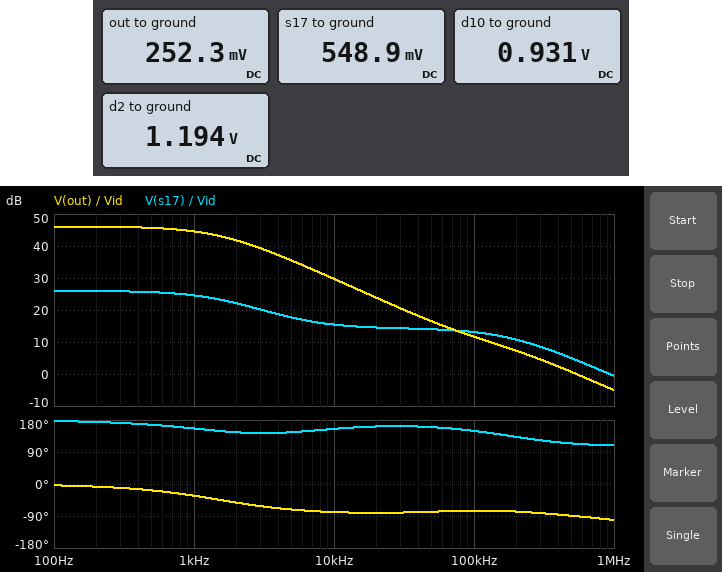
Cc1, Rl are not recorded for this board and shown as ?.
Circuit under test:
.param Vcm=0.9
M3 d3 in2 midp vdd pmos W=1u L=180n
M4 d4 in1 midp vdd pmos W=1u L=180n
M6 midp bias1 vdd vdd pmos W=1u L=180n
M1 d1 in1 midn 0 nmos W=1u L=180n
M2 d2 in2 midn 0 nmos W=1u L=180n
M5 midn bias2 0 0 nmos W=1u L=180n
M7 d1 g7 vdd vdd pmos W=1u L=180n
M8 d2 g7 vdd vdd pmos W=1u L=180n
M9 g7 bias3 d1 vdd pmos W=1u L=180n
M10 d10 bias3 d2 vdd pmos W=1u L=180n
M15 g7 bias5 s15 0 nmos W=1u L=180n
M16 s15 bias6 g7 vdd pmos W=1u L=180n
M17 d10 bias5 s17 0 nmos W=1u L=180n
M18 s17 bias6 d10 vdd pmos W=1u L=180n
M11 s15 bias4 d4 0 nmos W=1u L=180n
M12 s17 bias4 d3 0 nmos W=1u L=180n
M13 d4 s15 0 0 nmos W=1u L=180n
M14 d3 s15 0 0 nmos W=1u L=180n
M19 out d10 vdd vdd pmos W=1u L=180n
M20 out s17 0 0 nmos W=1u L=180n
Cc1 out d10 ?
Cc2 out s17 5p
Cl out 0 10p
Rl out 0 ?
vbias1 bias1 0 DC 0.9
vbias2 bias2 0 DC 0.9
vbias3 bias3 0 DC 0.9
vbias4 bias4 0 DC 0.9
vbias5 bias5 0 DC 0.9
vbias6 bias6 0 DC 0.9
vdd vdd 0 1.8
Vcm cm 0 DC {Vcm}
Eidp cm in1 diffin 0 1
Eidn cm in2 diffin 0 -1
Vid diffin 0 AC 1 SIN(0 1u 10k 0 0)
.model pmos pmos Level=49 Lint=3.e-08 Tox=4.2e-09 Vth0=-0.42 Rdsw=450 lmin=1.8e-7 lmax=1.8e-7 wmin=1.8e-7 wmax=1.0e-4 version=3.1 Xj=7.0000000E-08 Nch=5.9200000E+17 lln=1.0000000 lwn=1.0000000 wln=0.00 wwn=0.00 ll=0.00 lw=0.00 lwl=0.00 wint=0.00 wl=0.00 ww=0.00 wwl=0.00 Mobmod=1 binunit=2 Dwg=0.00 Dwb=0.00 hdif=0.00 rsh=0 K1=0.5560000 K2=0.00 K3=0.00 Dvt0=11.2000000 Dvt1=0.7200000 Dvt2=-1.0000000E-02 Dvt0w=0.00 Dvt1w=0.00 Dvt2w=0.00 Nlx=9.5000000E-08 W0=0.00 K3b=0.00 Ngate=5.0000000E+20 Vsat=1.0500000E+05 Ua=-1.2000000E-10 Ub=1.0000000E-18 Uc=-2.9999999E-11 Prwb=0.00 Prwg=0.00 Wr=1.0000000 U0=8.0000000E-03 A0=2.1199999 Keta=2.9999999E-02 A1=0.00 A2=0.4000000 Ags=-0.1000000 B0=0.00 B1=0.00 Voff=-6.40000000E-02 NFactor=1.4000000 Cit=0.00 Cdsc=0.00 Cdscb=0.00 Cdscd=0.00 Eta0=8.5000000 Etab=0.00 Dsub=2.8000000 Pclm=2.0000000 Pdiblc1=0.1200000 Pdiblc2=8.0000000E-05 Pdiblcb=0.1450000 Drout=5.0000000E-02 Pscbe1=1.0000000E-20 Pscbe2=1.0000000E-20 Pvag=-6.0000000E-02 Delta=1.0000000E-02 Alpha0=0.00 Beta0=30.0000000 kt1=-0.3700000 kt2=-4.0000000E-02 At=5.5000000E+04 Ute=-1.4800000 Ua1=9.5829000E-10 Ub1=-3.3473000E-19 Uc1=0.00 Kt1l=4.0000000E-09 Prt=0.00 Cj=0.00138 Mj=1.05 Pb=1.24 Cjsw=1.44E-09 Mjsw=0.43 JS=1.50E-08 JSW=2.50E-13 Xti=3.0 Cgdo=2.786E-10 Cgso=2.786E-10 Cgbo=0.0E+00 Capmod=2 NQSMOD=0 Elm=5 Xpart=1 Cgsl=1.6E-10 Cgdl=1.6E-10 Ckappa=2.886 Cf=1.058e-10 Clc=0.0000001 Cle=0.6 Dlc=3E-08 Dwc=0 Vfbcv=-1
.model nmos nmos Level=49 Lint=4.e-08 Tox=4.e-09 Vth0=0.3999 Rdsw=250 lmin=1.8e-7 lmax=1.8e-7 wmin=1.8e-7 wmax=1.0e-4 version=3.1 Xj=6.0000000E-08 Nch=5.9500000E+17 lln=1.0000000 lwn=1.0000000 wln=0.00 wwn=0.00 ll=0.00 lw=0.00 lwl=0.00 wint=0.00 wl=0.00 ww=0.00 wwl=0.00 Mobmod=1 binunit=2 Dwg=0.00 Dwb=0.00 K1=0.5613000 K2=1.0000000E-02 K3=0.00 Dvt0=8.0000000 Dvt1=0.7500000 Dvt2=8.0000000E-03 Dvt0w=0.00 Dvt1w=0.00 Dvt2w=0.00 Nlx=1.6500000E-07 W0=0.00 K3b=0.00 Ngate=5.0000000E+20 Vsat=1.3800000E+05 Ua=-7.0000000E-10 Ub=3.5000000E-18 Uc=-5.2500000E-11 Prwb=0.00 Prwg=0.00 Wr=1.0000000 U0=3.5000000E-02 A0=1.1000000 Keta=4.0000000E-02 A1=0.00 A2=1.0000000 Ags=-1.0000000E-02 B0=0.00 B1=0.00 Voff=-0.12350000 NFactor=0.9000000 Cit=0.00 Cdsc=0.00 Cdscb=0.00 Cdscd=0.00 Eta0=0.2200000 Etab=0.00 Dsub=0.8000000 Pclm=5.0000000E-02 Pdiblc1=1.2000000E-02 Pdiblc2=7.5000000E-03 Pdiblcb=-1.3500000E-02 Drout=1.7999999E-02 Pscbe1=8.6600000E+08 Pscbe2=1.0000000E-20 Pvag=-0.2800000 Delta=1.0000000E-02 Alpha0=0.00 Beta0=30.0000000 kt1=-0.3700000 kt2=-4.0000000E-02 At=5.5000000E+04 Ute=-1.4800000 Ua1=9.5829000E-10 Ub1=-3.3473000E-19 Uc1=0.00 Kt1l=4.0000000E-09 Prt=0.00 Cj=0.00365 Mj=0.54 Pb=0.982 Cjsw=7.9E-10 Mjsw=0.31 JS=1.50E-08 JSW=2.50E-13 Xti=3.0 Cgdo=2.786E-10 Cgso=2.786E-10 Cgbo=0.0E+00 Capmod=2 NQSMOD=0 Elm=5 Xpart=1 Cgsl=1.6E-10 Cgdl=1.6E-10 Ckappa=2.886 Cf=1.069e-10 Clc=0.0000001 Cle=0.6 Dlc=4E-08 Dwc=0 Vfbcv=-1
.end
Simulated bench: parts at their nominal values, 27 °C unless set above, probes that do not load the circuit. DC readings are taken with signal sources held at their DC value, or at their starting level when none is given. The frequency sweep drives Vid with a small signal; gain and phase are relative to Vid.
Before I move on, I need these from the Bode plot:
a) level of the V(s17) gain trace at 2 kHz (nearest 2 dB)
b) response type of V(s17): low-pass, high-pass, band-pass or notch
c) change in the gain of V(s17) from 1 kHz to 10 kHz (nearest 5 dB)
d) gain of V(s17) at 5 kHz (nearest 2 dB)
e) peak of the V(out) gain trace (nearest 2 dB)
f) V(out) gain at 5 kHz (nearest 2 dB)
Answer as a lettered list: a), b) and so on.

a) 22 dB
b) low-pass
c) -10 dB
d) 18 dB
e) 46 dB
f) 36 dB
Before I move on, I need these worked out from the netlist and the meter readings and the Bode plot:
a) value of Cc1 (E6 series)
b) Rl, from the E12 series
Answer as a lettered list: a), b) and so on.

a) 15 pF
b) 3.3 kΩ
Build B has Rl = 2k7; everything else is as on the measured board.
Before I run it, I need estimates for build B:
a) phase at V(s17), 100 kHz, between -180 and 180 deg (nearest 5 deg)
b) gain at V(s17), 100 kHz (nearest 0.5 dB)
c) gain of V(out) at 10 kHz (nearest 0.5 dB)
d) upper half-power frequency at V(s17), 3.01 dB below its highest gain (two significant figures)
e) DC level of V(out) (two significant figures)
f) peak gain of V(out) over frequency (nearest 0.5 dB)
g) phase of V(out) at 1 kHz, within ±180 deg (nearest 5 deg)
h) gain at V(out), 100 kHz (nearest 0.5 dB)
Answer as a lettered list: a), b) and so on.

a) 150 deg
b) 13.5 dB
c) 29.0 dB
d) 1.8 kHz
e) 210 mV
f) 44.5 dB
g) -30 deg
h) 10.5 dB
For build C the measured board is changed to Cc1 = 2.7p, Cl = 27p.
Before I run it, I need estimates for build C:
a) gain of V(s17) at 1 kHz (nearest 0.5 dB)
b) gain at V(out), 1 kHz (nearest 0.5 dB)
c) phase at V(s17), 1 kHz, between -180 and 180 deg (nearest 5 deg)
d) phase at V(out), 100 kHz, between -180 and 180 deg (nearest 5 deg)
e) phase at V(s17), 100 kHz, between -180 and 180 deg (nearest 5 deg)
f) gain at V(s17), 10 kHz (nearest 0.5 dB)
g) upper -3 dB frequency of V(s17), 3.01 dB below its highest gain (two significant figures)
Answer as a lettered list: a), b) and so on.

a) 26.0 dB
b) 46.0 dB
c) 170 deg
d) -90 deg
e) 125 deg
f) 20.0 dB
g) 5.9 kHz
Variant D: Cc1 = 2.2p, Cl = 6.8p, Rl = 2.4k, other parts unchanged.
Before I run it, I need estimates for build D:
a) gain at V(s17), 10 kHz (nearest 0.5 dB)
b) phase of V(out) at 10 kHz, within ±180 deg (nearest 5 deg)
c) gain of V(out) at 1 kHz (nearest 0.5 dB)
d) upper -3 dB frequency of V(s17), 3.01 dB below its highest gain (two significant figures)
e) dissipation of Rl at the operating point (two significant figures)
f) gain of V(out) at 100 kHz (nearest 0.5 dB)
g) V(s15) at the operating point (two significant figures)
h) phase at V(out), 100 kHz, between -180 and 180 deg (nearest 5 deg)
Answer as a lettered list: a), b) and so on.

a) 22.0 dB
b) -50 deg
c) 43.5 dB
d) 7.9 kHz
e) 15 µW
f) 21.5 dB
g) 550 mV
h) -85 deg
